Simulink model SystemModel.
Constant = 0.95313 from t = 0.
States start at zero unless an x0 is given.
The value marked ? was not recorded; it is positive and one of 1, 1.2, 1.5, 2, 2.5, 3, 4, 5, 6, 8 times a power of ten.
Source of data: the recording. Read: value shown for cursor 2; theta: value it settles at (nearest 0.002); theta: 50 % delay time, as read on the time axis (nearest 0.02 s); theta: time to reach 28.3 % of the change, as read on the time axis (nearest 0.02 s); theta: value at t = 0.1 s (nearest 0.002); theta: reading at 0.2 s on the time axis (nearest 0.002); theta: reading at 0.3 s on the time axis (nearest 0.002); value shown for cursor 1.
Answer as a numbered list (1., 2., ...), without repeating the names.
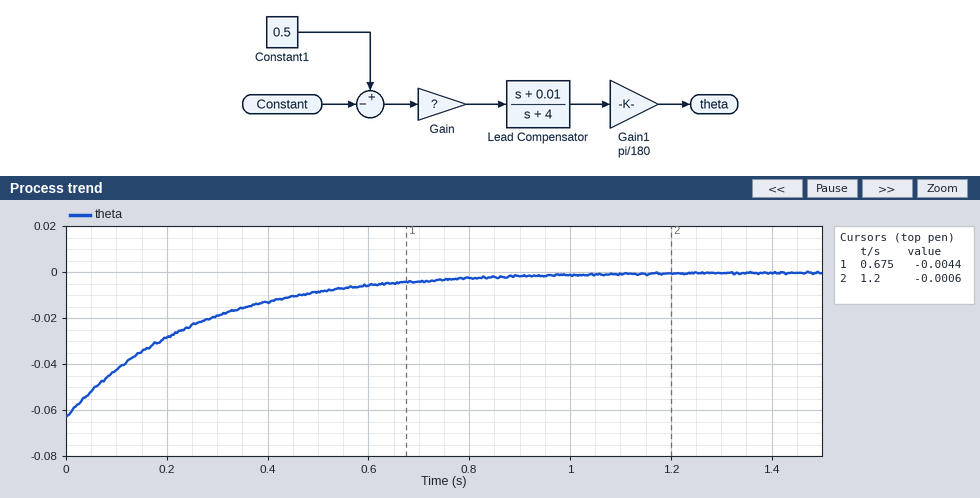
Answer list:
1. -0.0006
2. 0.000
3. 0.18 s
4. 0.08 s
5. -0.042
6. -0.028
7. -0.020
8. -0.0044
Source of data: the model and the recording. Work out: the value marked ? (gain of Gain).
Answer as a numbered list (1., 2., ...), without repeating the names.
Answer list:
1. 8
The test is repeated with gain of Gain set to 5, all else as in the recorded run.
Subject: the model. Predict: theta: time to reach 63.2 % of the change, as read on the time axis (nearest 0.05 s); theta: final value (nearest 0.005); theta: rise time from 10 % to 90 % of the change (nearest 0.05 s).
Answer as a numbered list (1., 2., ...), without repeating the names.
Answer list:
1. 0.25 s
2. 0.000
3. 0.55 s
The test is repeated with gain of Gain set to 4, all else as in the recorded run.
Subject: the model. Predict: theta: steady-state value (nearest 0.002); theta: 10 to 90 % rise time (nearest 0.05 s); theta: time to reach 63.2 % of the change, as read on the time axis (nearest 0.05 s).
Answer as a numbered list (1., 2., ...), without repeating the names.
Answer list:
1. 0.000
2. 0.55 s
3. 0.25 s
